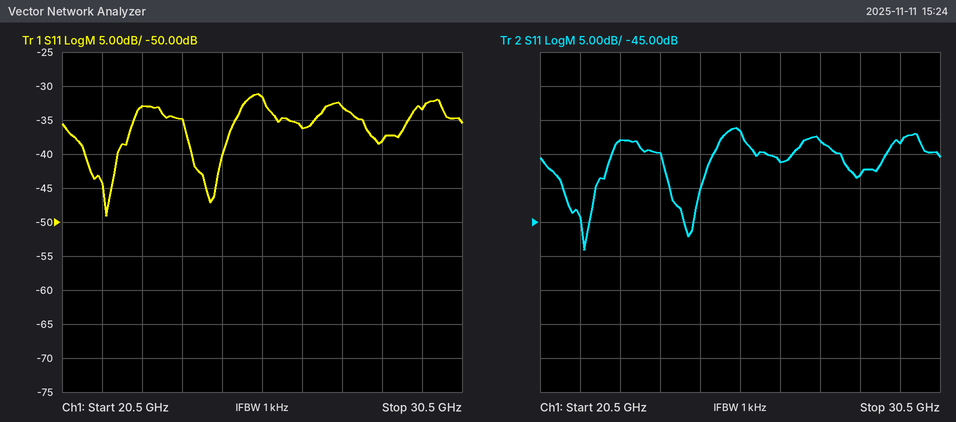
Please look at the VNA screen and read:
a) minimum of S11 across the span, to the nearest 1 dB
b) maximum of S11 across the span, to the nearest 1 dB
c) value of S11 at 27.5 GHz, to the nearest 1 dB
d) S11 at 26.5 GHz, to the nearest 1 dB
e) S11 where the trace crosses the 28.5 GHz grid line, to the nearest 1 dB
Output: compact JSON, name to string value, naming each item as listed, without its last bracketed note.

{"minimum of S11 across the span, to the nearest 1 dB": "-49 dB", "maximum of S11 across the span, to the nearest 1 dB": "-31 dB", "value of S11 at 27.5 GHz, to the nearest 1 dB": "-33 dB", "S11 at 26.5 GHz, to the nearest 1 dB": "-36 dB", "S11 where the trace crosses the 28.5 GHz grid line, to the nearest 1 dB": "-38 dB"}
